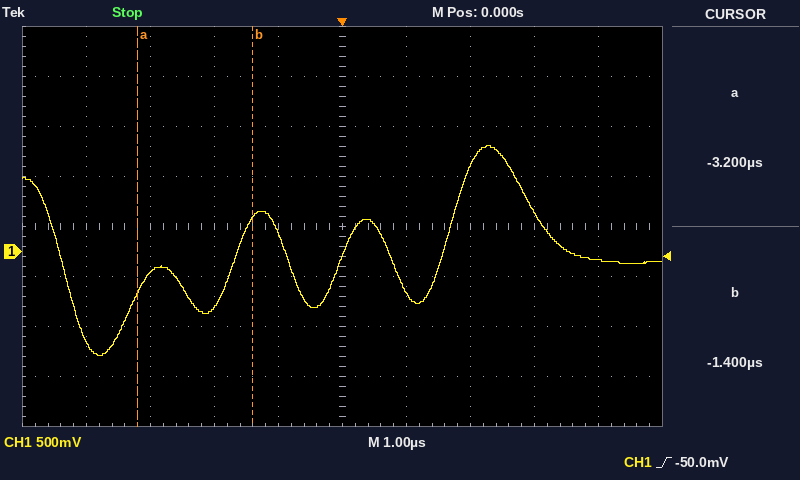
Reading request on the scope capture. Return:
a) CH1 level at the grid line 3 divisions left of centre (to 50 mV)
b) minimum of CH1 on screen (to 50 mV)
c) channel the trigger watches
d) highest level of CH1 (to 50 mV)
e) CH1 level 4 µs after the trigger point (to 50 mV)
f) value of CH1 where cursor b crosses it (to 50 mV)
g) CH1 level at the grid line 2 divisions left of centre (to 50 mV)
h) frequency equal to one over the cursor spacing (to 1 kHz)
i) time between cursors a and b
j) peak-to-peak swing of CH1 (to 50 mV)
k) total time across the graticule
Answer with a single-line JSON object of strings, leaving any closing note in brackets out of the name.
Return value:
{"CH1 level at the grid line 3 divisions left of centre": "-200 mV", "minimum of CH1 on screen": "-1.05 V", "channel the trigger watches": "CH1", "highest level of CH1": "1.05 V", "CH1 level 4 µs after the trigger point": "-100 mV", "value of CH1 where cursor b crosses it": "350 mV", "CH1 level at the grid line 2 divisions left of centre": "-550 mV", "frequency equal to one over the cursor spacing": "556 kHz", "time between cursors a and b": "1.8 µs", "peak-to-peak swing of CH1": "2.10 V", "total time across the graticule": "10 µs"}
